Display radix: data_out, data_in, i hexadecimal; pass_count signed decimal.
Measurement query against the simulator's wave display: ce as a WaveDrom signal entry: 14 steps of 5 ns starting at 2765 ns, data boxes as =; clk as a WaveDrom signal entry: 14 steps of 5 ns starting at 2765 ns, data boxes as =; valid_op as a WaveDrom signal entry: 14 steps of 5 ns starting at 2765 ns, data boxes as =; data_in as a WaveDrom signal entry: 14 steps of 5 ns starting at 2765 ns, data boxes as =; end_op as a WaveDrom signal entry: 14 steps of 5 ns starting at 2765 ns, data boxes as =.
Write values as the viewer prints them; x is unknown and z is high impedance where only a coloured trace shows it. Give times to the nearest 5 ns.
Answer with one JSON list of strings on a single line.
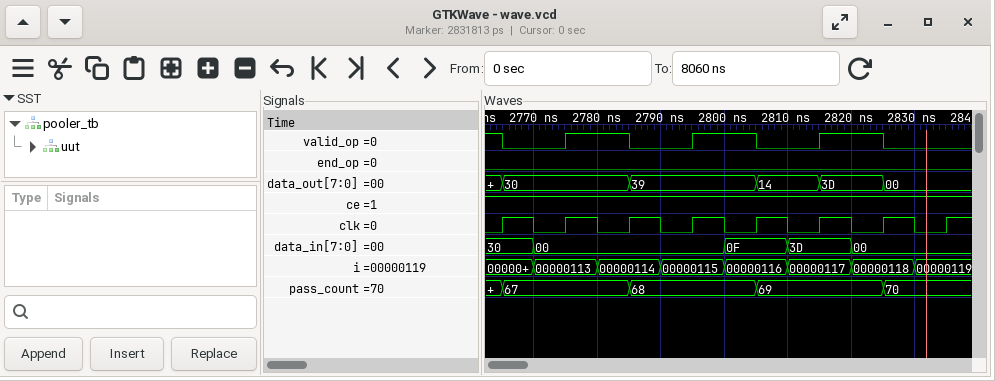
["{name: 'ce', wave: '1.............'}", "{name: 'clk', wave: '10101010101010'}", "{name: 'valid_op', wave: '0.1.0.1.0.1.0.'}", "{name: 'data_in', wave: '==.....=.=.=..', data: '30 00 0F 3D 00'}", "{name: 'end_op', wave: '0.............'}"]
